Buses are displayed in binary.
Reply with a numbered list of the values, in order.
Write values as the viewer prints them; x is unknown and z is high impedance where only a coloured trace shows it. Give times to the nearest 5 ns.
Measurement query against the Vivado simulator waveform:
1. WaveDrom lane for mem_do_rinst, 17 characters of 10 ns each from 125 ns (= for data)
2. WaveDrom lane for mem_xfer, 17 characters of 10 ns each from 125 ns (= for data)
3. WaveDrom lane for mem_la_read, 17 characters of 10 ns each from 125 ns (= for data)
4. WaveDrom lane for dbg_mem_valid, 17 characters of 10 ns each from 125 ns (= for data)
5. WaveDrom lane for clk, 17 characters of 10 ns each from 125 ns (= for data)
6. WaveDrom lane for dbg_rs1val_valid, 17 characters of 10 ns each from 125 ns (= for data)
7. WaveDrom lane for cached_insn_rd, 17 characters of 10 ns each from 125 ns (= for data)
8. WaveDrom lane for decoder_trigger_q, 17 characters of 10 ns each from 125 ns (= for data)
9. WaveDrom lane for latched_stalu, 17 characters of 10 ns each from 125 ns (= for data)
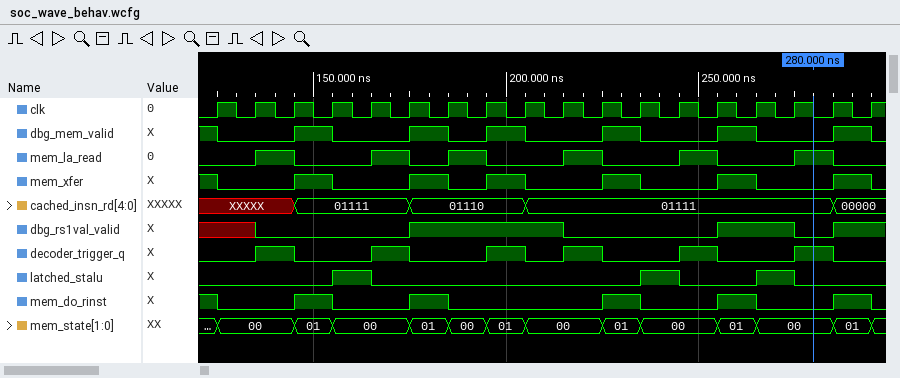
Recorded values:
1. {name: 'mem_do_rinst', wave: '0.10.10...10.10.1'}
2. {name: 'mem_xfer', wave: '0.10.1010.10.10.1'}
3. {name: 'mem_la_read', wave: '010.1010.10.10.10'}
4. {name: 'dbg_mem_valid', wave: '0.10.1010.10.10.1'}
5. {name: 'clk', wave: 'p................'}
6. {name: 'dbg_rs1val_valid', wave: 'x0...1...0...1.01'}
7. {name: 'cached_insn_rd', wave: 'x.=..=..=.......=', data: '01111 01110 01111 00000'}
8. {name: 'decoder_trigger_q', wave: '010.10.1010.10.10'}
9. {name: 'latched_stalu', wave: '0..10......10.10.'}
